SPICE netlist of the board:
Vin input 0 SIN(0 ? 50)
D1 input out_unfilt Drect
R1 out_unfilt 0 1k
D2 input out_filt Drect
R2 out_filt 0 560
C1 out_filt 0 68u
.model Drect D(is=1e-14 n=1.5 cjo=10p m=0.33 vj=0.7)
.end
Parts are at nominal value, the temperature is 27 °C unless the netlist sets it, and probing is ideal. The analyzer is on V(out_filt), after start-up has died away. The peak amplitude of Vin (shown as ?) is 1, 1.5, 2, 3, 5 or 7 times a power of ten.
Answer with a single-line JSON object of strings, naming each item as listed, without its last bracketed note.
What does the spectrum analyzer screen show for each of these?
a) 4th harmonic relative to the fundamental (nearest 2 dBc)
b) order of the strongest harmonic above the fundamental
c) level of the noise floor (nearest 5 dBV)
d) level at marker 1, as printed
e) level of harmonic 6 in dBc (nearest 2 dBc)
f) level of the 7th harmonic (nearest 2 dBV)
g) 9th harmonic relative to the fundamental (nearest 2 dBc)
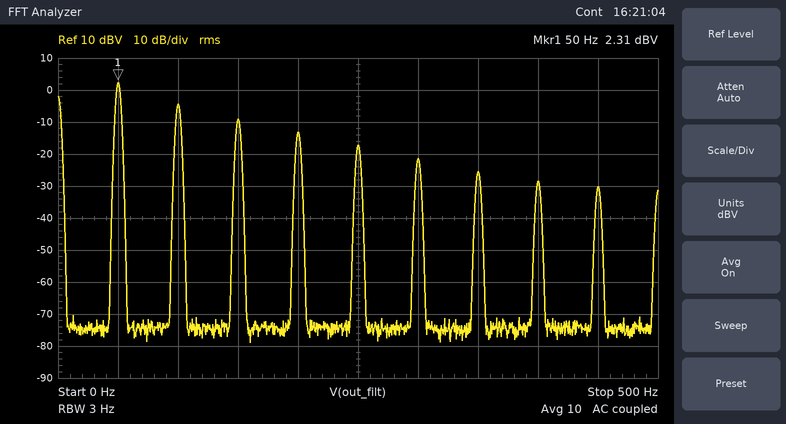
{"4th harmonic relative to the fundamental": "-16 dBc", "order of the strongest harmonic above the fundamental": "2", "level of the noise floor": "-75 dBV", "level at marker 1, as printed": "2.31 dBV", "level of harmonic 6 in dBc": "-24 dBc", "level of the 7th harmonic": "-26 dBV", "9th harmonic relative to the fundamental": "-32 dBc"}
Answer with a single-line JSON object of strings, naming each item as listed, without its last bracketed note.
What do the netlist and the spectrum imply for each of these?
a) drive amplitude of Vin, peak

{"drive amplitude of Vin, peak": "15 V"}
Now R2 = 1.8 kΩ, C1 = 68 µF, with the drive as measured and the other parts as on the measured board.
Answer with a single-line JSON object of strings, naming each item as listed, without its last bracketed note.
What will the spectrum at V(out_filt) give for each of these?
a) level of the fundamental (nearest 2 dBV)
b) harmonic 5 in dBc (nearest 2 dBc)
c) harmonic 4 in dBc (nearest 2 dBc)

{"level of the fundamental": "-6 dBV", "harmonic 5 in dBc": "-16 dBc", "harmonic 4 in dBc": "-14 dBc"}
